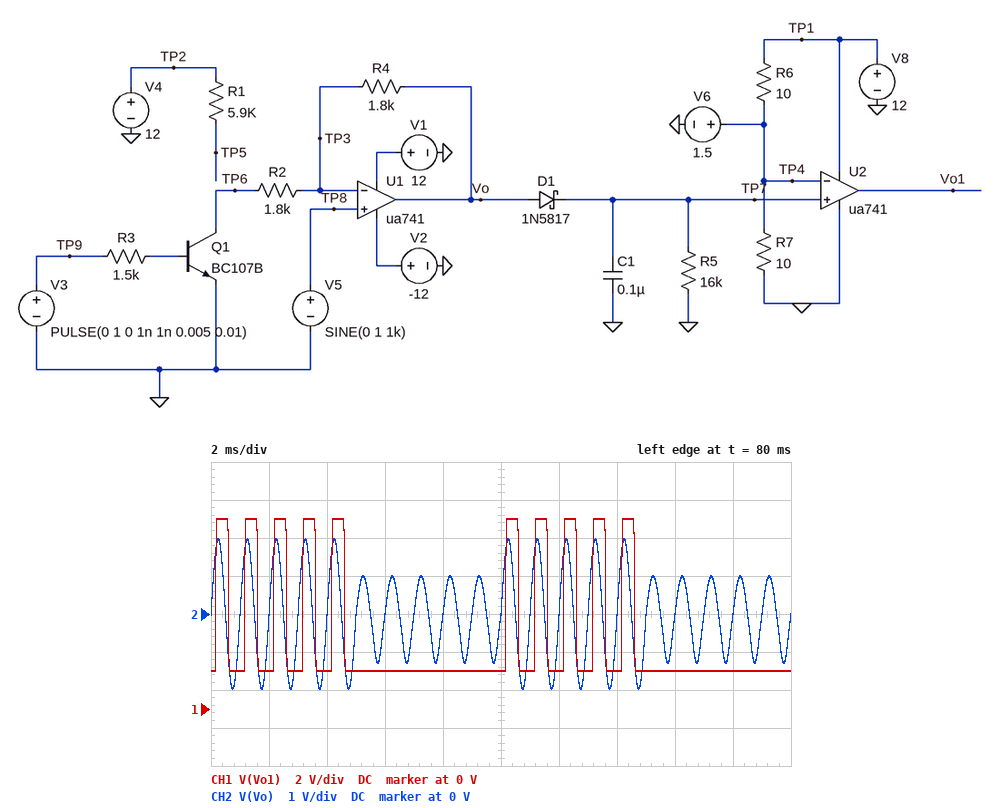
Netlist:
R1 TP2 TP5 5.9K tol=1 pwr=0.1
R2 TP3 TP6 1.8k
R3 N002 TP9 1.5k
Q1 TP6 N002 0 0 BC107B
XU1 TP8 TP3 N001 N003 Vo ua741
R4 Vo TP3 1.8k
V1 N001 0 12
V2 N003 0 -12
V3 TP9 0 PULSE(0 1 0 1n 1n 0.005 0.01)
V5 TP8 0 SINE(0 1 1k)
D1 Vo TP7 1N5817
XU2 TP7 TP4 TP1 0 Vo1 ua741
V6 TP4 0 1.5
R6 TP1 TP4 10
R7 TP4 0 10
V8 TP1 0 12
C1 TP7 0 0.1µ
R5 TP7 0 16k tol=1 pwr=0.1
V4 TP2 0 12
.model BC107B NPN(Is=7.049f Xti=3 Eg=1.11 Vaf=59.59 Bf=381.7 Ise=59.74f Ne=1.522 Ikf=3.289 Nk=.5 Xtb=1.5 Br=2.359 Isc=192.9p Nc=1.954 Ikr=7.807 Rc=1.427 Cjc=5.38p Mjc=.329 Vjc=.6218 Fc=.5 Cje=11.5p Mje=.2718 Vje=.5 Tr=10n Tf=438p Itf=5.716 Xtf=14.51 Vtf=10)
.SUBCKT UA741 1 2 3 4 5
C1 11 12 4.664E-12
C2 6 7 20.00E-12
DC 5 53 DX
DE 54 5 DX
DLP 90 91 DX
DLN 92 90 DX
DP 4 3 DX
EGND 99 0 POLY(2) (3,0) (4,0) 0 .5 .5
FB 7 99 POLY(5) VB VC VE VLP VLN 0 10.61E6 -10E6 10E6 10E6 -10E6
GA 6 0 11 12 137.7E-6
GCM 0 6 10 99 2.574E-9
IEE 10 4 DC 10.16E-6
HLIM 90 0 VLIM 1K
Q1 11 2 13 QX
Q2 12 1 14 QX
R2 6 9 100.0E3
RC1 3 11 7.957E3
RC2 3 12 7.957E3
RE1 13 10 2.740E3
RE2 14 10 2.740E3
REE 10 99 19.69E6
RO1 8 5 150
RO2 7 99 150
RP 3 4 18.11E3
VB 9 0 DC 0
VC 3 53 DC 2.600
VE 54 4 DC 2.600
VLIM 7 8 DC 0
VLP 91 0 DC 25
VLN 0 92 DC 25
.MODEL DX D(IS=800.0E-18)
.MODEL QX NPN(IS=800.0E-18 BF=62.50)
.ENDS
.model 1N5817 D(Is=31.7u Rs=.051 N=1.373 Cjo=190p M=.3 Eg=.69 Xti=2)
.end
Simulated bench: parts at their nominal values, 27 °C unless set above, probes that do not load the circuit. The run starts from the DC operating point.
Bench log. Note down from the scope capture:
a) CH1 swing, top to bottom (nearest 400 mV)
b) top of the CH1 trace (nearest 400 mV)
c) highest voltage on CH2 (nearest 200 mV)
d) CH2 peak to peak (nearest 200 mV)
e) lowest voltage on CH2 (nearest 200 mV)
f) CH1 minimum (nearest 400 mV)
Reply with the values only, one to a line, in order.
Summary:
8.0 V
10.0 V
2.0 V
4.0 V
-2.0 V
2.0 V
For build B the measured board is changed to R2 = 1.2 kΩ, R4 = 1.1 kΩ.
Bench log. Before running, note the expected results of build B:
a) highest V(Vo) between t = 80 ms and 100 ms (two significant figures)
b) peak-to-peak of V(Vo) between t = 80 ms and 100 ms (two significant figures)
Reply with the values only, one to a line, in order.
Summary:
1.9 V
3.7 V
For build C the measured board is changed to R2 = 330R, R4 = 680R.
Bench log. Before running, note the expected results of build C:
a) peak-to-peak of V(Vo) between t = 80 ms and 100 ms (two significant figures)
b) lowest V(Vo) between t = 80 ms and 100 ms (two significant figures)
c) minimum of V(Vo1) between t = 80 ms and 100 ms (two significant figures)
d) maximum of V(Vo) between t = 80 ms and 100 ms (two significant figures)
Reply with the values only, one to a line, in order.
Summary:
5.0 V
-2.1 V
2.0 V
2.9 V
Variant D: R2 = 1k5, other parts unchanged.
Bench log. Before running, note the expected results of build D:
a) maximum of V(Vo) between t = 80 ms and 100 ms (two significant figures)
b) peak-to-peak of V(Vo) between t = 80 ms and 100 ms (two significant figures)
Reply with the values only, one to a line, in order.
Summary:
2.2 V
4.3 V
